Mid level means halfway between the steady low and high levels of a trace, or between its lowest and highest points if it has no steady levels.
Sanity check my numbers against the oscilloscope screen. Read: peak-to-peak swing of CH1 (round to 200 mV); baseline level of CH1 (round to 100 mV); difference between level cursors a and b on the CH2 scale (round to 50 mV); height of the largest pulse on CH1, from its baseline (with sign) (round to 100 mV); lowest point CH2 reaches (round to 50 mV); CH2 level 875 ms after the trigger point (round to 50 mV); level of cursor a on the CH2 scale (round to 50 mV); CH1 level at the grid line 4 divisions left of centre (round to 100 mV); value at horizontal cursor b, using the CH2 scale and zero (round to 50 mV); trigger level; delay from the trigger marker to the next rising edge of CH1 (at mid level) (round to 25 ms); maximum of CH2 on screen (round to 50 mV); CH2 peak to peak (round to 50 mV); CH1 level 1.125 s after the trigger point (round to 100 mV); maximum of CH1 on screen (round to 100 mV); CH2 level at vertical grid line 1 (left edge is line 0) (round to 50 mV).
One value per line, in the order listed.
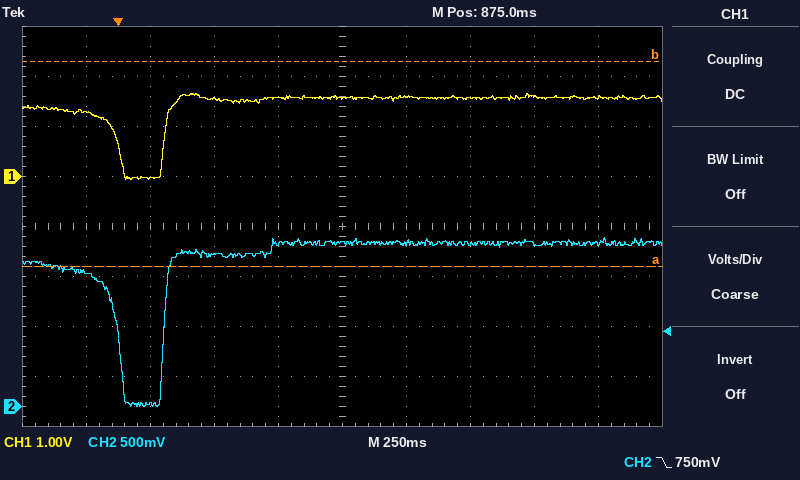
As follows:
1.8 V
1.6 V
2.05 V
-1.6 V
0 mV
1.65 V
1.40 V
1.3 V
3.45 V
750 mV
175 ms
1.70 V
1.70 V
1.6 V
1.7 V
1.35 V
